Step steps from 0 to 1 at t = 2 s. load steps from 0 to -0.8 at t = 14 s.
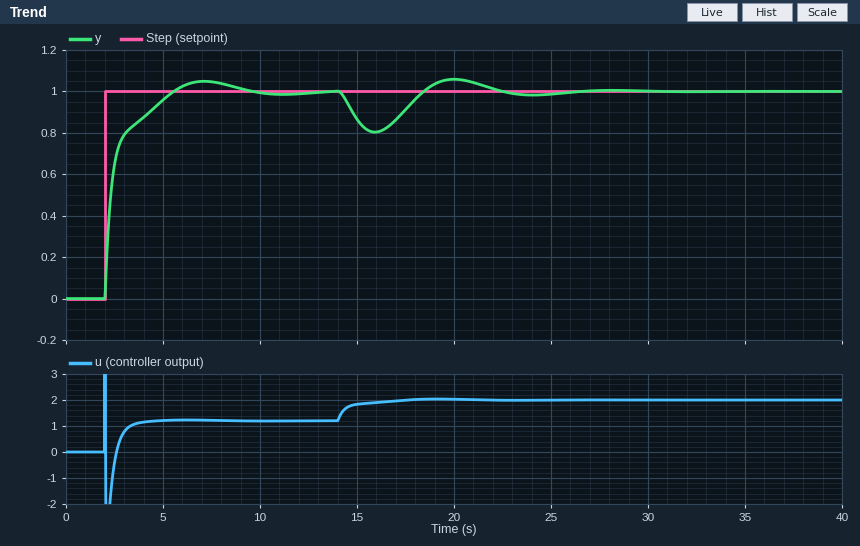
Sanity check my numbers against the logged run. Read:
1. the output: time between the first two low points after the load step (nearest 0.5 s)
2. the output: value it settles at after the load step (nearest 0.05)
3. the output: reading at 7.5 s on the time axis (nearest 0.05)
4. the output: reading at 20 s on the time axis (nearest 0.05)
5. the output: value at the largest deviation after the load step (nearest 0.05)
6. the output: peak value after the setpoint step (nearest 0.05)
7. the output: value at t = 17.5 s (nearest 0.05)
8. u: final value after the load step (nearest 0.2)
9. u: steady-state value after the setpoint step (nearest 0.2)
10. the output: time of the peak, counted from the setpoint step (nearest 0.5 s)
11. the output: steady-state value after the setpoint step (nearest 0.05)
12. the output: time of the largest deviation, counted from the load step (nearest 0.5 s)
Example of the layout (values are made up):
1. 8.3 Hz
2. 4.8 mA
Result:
1. 8.0 s
2. 1.00
3. 1.05
4. 1.05
5. 0.80
6. 1.05
7. 0.90
8. 2.0
9. 1.2
10. 5.0 s
11. 1.00
12. 2.0 s
